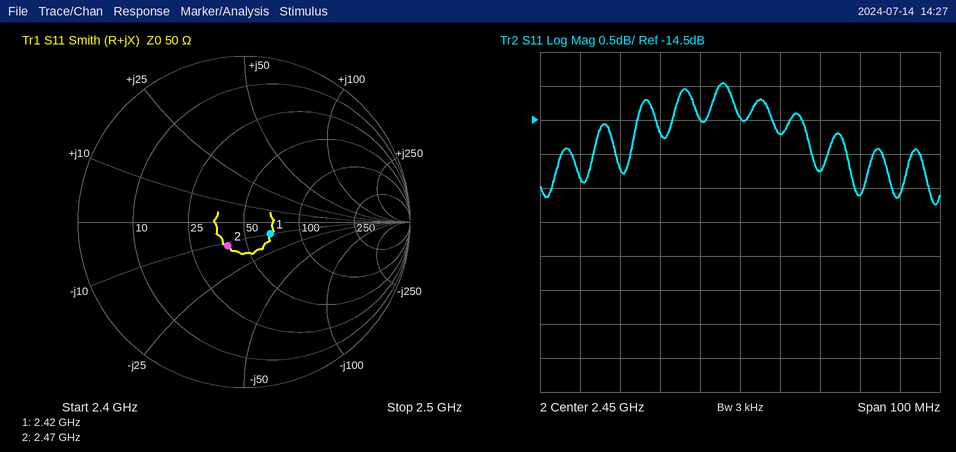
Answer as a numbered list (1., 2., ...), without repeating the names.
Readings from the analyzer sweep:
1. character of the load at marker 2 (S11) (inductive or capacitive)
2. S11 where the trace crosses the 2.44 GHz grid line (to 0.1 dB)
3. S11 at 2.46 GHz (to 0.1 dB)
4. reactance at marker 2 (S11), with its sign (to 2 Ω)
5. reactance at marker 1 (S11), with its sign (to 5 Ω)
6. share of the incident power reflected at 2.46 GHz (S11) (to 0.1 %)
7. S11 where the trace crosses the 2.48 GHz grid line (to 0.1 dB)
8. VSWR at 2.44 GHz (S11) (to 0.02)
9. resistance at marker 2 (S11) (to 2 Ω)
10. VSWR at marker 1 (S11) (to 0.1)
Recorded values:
1. capacitive
2. -14.5 dB
3. -14.7 dB
4. -12 Ω
5. -10 Ω
6. 3.4 %
7. -15.6 dB
8. 1.46
9. 40 Ω
10. 1.4
